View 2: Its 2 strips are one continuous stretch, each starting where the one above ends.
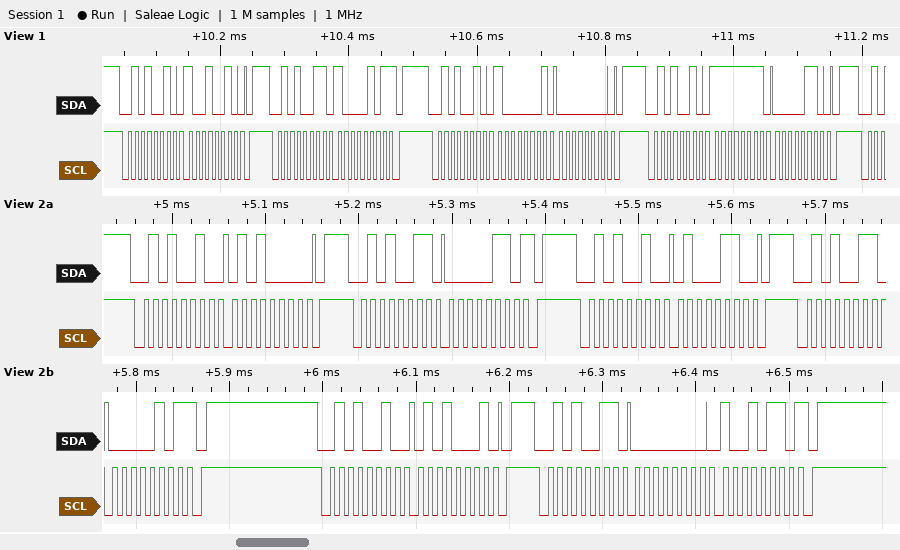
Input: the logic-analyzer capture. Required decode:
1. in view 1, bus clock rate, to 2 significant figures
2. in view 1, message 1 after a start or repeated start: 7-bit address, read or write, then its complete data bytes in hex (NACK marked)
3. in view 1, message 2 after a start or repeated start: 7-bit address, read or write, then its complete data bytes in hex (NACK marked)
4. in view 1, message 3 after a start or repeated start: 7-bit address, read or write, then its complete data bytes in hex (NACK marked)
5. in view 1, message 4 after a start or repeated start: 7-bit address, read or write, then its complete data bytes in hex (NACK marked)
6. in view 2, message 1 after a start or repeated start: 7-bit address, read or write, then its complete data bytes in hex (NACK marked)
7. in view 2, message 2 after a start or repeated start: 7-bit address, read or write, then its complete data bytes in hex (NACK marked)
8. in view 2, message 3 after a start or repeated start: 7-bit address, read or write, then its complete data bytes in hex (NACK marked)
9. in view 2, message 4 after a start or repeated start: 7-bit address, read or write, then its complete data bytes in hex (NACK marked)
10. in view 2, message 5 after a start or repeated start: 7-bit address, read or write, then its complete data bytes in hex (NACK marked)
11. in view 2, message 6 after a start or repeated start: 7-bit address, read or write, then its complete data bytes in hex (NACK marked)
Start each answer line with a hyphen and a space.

- 100 kHz
- 0x29 write: 92
- 0x29 read: 85 NACK
- 0x29 write: 81 00
- 0x29 write: FF 06
- 0x29 write: 50
- 0x29 read: 06 NACK
- 0x29 write: 46
- 0x29 read: 05 NACK
- 0x29 write: 51
- 0x29 read: 00 96 NACK
